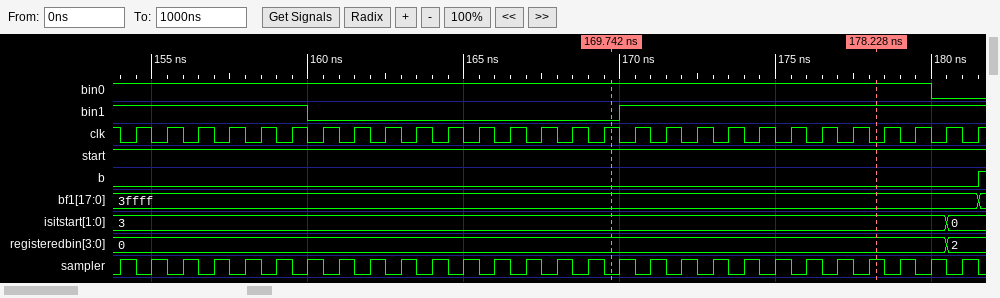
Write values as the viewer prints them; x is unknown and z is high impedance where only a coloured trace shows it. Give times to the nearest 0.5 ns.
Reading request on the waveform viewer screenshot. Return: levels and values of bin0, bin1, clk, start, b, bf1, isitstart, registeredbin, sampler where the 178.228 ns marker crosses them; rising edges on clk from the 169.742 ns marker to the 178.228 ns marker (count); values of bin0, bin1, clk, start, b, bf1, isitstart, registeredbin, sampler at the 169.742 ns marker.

bin0=1, bin1=1, clk=0, start=1, b=0, bf1=3ffff, isitstart=3, registeredbin=0, sampler=1
8
bin0=1, bin1=0, clk=1, start=1, b=0, bf1=3ffff, isitstart=3, registeredbin=0, sampler=0
